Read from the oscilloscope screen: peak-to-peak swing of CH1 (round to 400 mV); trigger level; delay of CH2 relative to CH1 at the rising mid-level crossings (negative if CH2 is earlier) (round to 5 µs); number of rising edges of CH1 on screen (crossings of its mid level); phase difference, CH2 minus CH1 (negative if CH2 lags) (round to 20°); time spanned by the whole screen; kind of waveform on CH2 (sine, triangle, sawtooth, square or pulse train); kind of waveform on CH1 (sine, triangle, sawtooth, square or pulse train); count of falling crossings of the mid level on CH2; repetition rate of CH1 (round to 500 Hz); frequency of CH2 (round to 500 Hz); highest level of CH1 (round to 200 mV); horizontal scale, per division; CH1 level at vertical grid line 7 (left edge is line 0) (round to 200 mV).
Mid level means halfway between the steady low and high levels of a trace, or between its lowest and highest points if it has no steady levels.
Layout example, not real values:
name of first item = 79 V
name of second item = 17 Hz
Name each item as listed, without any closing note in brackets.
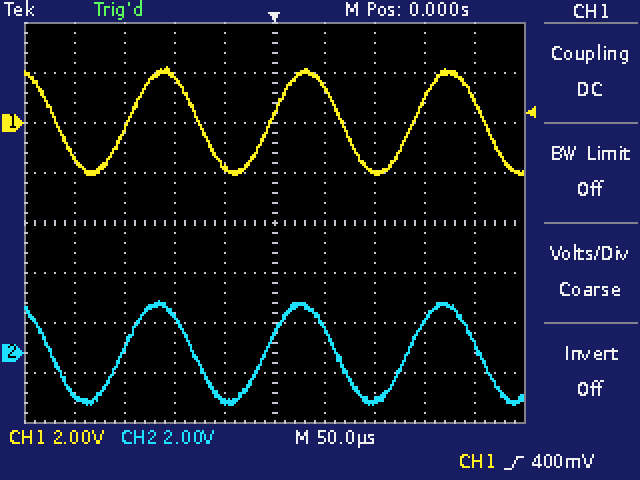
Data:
peak-to-peak swing of CH1 = 4.4 V
trigger level = 400 mV
delay of CH2 relative to CH1 at the rising mid-level crossings (negative if CH2 is earlier) = -5 µs
number of rising edges of CH1 on screen = 3
phase difference, CH2 minus CH1 (negative if CH2 lags) = +20°
time spanned by the whole screen = 500 µs
kind of waveform on CH2 = sine
kind of waveform on CH1 = sine
count of falling crossings of the mid level on CH2 = 4
repetition rate of CH1 = 7.0 kHz
frequency of CH2 = 7.0 kHz
highest level of CH1 = 2.2 V
horizontal scale, per division = 50 µs
CH1 level at vertical grid line 7 (left edge is line 0) = -2.0 V
